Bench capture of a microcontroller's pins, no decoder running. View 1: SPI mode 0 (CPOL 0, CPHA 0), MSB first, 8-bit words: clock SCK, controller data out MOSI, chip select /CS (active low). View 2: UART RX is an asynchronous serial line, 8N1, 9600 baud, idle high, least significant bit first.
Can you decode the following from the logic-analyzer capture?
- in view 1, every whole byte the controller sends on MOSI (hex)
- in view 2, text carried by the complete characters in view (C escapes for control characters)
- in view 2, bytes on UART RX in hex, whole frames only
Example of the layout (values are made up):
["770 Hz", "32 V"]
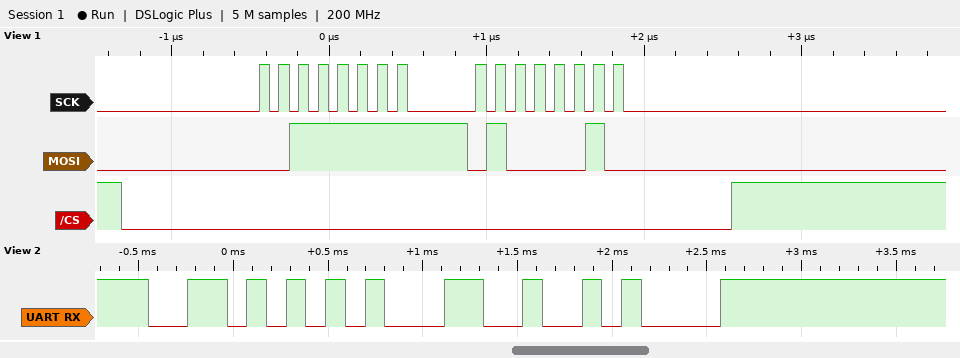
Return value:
["3F 42", "\"V1\\n\"", "0x56 0x31 0x0A"]
